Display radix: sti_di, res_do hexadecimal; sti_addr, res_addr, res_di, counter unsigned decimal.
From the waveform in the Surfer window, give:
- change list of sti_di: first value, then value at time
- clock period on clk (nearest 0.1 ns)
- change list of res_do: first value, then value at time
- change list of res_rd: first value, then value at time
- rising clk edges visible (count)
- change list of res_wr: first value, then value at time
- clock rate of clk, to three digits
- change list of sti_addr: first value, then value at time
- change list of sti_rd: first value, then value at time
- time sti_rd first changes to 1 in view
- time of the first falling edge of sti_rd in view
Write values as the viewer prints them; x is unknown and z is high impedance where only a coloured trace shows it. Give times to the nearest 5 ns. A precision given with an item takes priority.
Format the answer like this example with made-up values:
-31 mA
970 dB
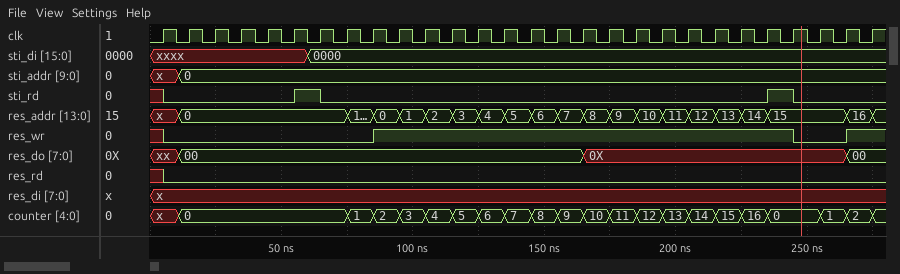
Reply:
xxxx, 0000 at 60 ns
10 ns
xx, 00 at 10 ns, 0X at 165 ns, 00 at 265 ns
x, 0 at 5 ns
28
x, 0 at 5 ns, 1 at 85 ns, 0 at 245 ns, 1 at 265 ns
100 MHz
x, 0 at 10 ns
x, 0 at 5 ns, 1 at 55 ns, 0 at 65 ns, 1 at 235 ns, 0 at 245 ns
55 ns
65 ns
